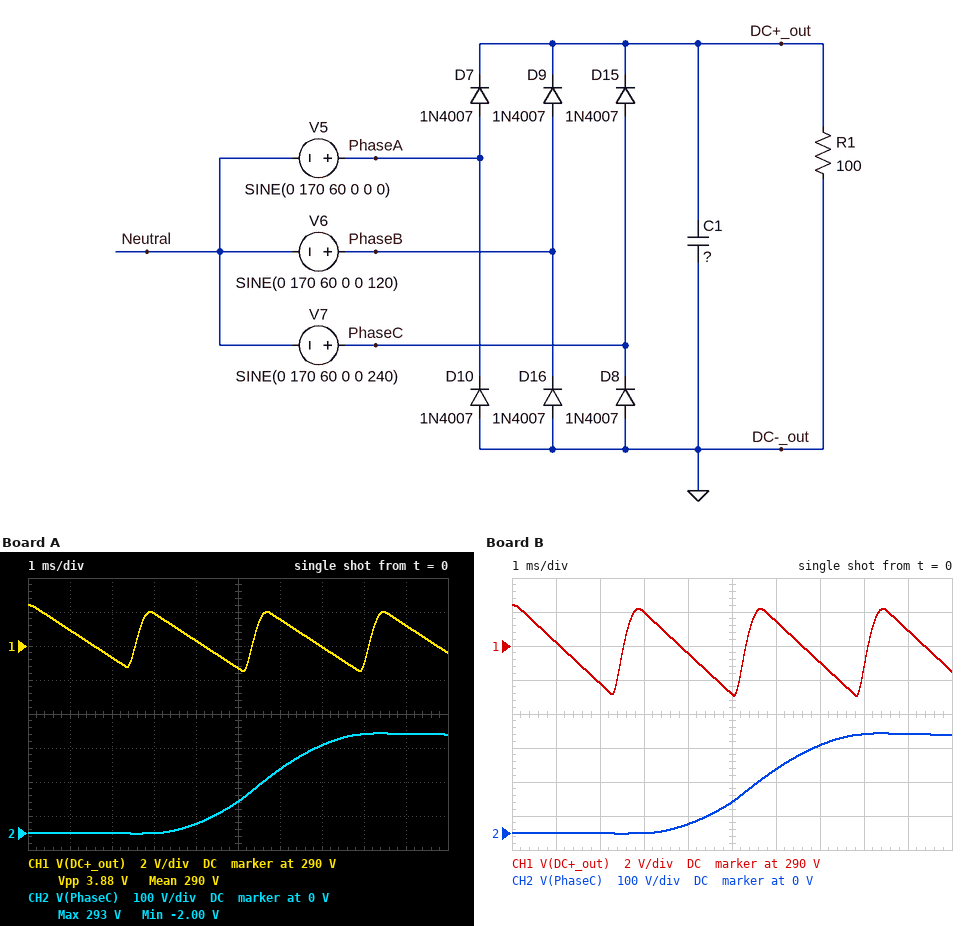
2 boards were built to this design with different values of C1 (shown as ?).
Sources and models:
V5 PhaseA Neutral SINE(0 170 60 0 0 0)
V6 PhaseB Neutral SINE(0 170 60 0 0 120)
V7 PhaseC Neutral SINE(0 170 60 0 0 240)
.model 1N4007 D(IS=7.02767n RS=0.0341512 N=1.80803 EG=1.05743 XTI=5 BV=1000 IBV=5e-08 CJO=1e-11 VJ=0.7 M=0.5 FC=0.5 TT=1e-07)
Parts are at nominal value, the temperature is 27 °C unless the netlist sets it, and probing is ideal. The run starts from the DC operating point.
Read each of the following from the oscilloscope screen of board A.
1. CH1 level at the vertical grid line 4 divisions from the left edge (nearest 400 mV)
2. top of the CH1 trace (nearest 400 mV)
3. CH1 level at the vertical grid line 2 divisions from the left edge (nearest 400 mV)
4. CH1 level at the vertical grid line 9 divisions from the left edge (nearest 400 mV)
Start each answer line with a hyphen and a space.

- 290.4 V
- 292.4 V
- 289.2 V
- 291.2 V
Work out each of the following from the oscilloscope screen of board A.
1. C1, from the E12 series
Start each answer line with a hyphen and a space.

- 1.8 mF
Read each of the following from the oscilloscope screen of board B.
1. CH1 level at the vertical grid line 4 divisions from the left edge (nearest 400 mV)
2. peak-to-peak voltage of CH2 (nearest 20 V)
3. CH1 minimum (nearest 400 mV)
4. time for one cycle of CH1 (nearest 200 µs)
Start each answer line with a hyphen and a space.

- 289.6 V
- 300 V
- 287.2 V
- 2.8 ms
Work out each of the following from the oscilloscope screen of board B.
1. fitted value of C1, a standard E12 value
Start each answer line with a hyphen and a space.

- 1.2 mF
